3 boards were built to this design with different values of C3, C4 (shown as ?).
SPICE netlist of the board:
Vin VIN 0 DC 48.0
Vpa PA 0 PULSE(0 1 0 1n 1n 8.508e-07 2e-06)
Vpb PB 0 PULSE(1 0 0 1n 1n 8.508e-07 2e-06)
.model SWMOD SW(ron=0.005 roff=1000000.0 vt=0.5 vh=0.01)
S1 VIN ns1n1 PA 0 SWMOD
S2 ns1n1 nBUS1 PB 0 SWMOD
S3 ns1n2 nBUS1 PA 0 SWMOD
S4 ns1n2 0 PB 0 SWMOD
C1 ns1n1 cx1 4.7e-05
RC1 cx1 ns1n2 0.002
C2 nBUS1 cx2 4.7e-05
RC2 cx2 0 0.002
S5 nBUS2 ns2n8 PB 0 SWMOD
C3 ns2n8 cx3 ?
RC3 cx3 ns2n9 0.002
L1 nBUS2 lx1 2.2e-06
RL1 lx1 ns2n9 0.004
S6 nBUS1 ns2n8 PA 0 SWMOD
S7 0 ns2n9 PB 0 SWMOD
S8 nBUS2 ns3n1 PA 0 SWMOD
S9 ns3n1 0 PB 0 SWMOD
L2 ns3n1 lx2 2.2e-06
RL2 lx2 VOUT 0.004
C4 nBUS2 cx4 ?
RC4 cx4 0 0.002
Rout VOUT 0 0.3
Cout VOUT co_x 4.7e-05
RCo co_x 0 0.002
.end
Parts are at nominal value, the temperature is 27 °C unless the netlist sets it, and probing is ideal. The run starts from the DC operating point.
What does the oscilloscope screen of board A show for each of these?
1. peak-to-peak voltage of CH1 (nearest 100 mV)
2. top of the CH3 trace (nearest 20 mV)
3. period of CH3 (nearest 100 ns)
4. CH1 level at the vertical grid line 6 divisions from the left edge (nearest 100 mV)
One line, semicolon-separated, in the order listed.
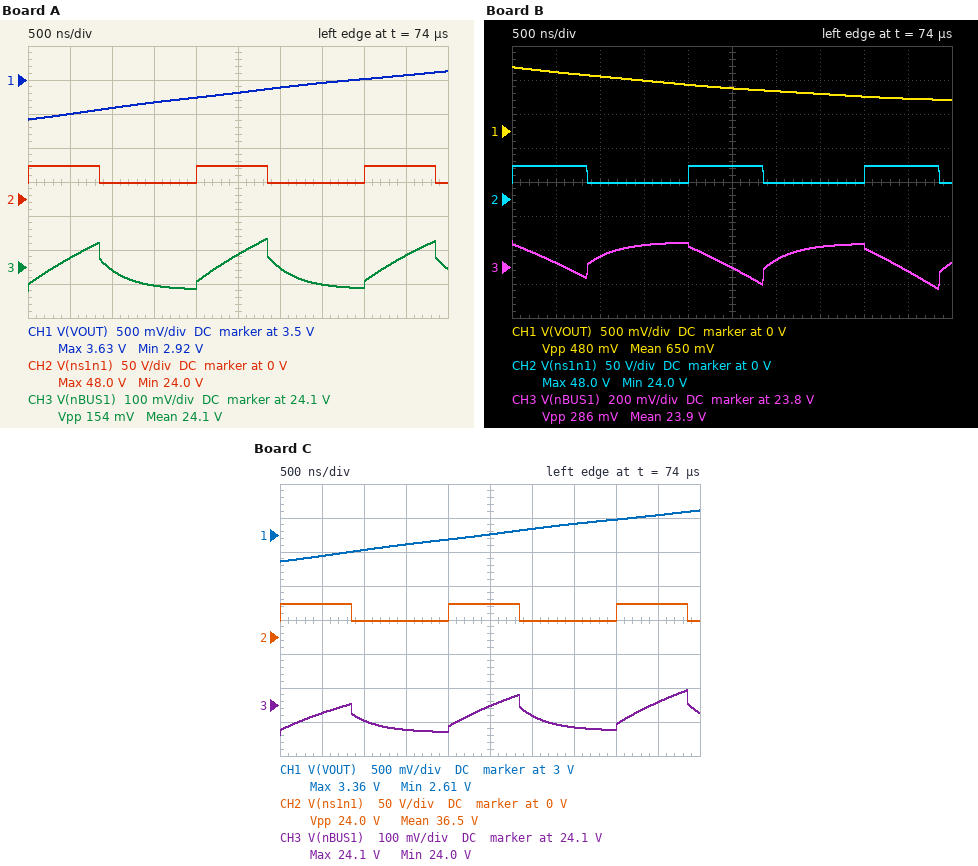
700 mV; 24.18 V; 2.0 µs; 3.4 V
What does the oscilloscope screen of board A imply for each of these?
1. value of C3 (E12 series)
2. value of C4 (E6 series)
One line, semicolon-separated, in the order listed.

18 µF; 33 µF
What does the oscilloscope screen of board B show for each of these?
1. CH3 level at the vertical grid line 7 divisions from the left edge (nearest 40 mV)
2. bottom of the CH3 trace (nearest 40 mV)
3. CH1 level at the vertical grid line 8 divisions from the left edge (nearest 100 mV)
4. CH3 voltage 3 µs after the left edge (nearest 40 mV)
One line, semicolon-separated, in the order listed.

23.92 V; 23.68 V; 500 mV; 23.84 V
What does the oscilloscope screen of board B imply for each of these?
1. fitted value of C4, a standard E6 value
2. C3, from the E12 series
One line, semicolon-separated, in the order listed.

68 µF; 39 µF
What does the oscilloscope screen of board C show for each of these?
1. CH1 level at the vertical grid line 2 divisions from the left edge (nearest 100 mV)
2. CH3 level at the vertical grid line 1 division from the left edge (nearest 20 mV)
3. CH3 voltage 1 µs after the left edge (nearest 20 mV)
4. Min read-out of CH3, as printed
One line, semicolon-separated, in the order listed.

2.8 V; 24.08 V; 24.06 V; 24.0 V
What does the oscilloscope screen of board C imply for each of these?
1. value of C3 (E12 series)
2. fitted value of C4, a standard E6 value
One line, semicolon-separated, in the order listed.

39 µF; 15 µF
